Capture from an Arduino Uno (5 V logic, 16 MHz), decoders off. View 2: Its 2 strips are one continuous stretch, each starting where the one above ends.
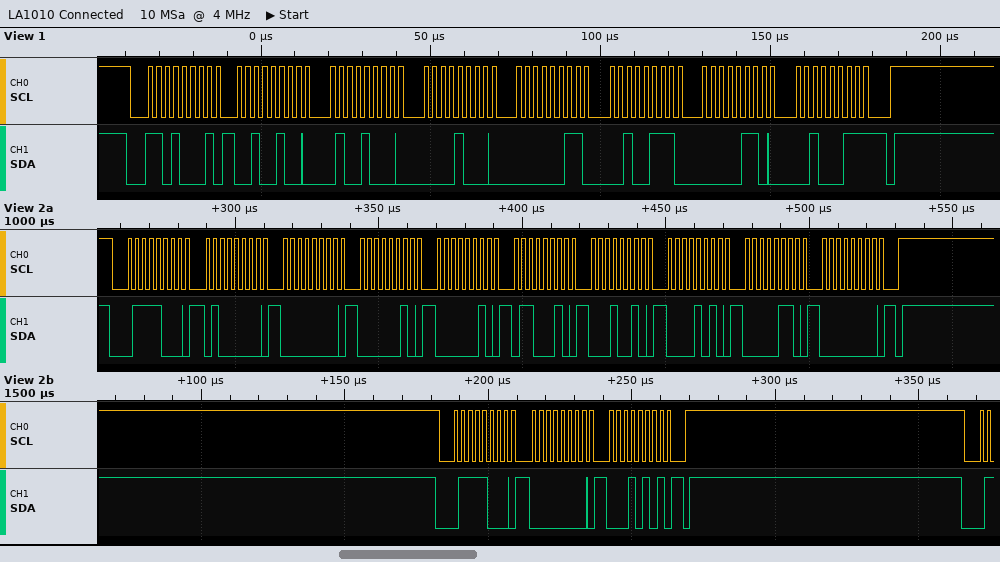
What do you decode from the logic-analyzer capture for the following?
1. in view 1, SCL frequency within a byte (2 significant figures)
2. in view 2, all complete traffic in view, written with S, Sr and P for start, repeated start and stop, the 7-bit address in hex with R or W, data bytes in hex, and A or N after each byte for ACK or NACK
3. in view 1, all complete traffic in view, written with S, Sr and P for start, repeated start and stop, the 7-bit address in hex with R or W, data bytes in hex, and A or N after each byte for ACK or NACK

400 kHz
S 3CW A 40 A 00 A 02 A 02 A 62 A 12 A 0A A 06 A 00 A P S 3CW A 00 A 15 A P
S 68R A 24 A 48 A 08 A 03 A 27 A 06 A 23 N P
